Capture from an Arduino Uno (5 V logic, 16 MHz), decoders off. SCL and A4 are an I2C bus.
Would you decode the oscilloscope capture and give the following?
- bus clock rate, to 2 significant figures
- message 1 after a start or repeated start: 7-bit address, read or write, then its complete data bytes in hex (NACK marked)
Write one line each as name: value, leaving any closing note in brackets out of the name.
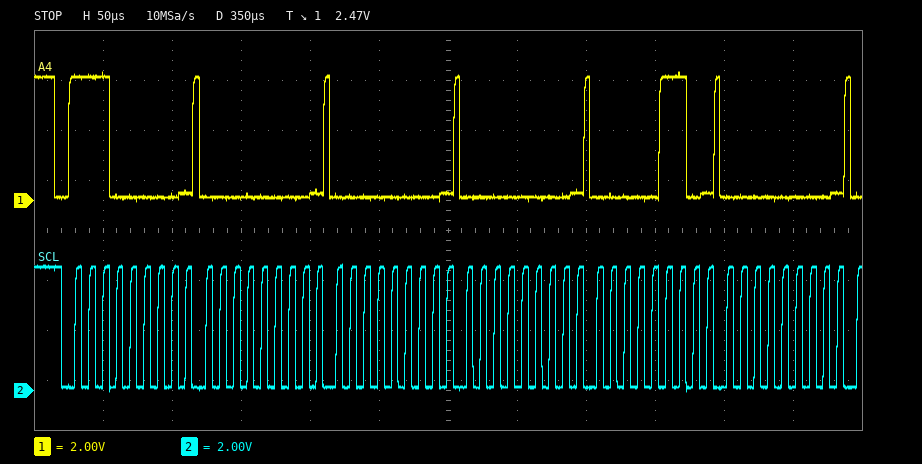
bus clock rate, to 2 significant figures: 100 kHz
message 1 after a start or repeated start: 7-bit address, read or write, then its complete data bytes in hex: 0x70 write: 00 00 00 06 00
